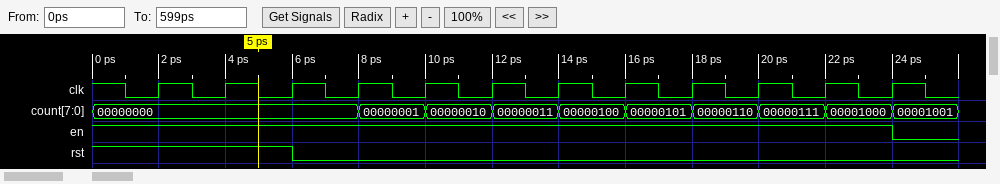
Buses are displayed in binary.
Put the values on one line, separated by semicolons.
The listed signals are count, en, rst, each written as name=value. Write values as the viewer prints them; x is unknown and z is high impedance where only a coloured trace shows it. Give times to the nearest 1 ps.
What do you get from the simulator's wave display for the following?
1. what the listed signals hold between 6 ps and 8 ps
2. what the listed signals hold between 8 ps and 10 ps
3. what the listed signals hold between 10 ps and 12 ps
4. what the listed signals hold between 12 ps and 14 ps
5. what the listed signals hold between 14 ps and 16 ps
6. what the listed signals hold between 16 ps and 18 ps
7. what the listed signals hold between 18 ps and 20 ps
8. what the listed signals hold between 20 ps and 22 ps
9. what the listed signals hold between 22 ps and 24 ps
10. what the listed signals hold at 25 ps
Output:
count=00000000, en=1, rst=0; count=00000001, en=1, rst=0; count=00000010, en=1, rst=0; count=00000011, en=1, rst=0; count=00000100, en=1, rst=0; count=00000101, en=1, rst=0; count=00000110, en=1, rst=0; count=00000111, en=1, rst=0; count=00001000, en=1, rst=0; count=00001001, en=0, rst=0
